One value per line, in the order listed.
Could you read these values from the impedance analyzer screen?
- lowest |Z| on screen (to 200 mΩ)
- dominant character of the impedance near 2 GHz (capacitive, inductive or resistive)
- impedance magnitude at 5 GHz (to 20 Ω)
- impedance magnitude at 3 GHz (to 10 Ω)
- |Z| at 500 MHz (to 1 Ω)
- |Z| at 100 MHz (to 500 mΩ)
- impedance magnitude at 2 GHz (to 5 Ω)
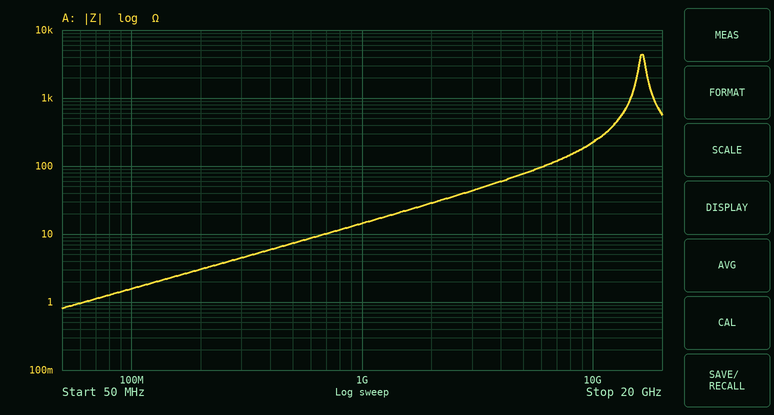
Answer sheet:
800 mΩ
inductive
80 Ω
40 Ω
7 Ω
1.5 Ω
30 Ω
